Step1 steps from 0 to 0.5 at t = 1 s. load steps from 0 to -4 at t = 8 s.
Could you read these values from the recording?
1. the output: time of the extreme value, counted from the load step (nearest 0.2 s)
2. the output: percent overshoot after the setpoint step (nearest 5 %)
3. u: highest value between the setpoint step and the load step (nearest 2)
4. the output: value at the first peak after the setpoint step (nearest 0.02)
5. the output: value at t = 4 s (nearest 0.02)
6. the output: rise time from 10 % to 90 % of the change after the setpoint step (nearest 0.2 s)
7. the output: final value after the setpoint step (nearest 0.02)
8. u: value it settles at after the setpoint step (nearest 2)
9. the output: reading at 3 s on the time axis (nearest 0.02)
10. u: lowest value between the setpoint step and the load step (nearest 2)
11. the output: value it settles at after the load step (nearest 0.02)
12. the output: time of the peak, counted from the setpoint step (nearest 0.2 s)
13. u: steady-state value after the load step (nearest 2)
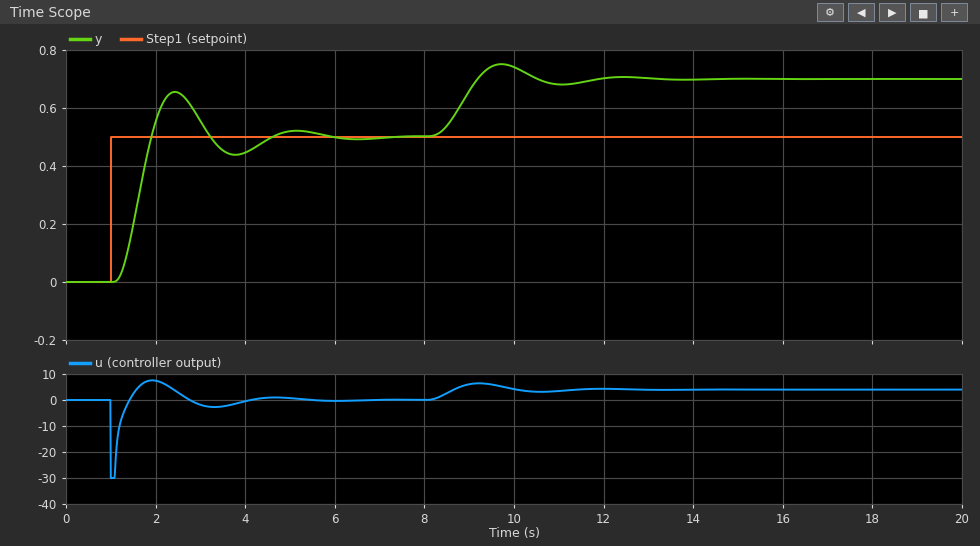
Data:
1.8 s
30 %
8
0.66
0.44
0.6 s
0.50
0
0.56
-30
0.70
1.4 s
4
